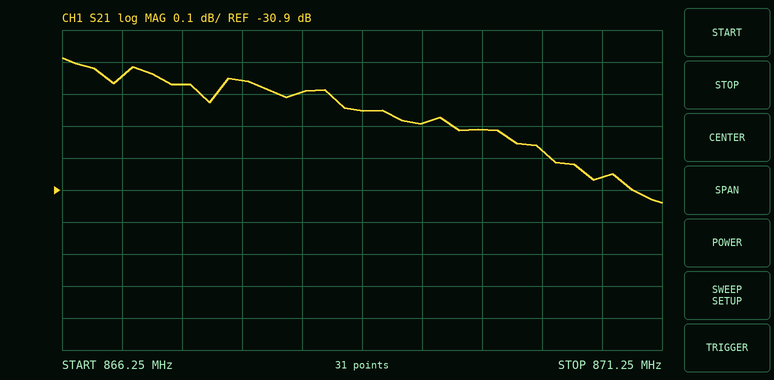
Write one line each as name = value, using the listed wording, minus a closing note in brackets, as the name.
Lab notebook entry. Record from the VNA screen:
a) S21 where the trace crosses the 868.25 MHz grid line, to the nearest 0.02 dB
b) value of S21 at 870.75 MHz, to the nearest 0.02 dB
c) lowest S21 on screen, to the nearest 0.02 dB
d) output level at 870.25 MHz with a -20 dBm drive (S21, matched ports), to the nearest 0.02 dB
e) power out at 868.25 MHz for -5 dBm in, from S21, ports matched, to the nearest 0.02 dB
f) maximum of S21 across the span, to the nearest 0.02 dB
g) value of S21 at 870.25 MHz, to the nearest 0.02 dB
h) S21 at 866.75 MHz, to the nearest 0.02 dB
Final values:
S21 where the trace crosses the 868.25 MHz grid line, to the nearest 0.02 dB = -30.60 dB
value of S21 at 870.75 MHz, to the nearest 0.02 dB = -30.86 dB
lowest S21 on screen, to the nearest 0.02 dB = -30.94 dB
output level at 870.25 MHz with a -20 dBm drive (S21, matched ports), to the nearest 0.02 dB = -50.78 dBm
power out at 868.25 MHz for -5 dBm in, from S21, ports matched, to the nearest 0.02 dB = -35.60 dBm
maximum of S21 across the span, to the nearest 0.02 dB = -30.48 dB
value of S21 at 870.25 MHz, to the nearest 0.02 dB = -30.78 dB
S21 at 866.75 MHz, to the nearest 0.02 dB = -30.54 dB
